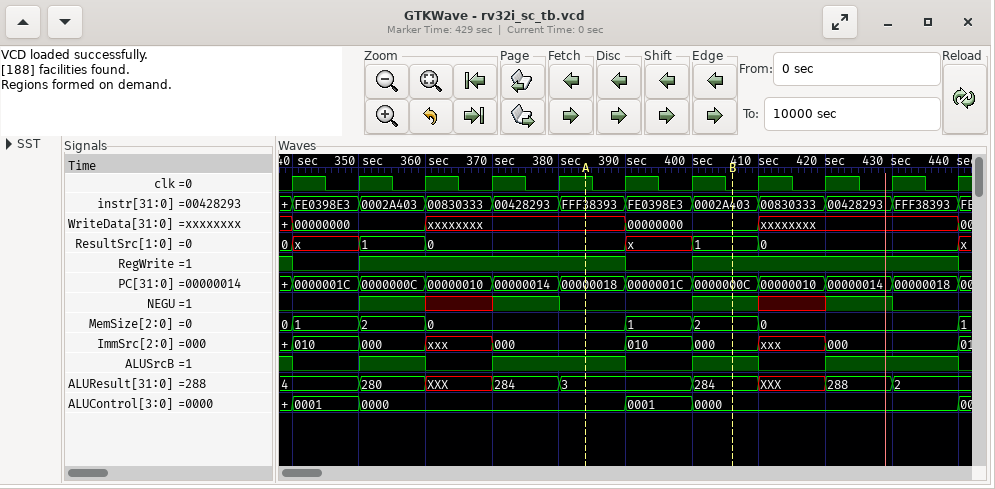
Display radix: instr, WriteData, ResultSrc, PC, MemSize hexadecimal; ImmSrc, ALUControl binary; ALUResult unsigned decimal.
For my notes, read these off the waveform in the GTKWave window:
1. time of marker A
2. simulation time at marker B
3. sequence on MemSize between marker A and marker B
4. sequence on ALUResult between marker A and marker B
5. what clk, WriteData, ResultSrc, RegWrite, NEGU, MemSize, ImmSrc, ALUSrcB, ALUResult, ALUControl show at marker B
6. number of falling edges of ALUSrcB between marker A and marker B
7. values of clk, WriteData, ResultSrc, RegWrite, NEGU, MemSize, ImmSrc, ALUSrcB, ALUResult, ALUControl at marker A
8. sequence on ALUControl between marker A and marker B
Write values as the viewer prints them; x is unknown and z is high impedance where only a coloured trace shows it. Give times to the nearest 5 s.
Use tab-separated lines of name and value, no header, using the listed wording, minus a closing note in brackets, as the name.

time of marker A	385 s
simulation time at marker B	405 s
sequence on MemSize between marker A and marker B	0, 1, 2
sequence on ALUResult between marker A and marker B	3, 284
what clk, WriteData, ResultSrc, RegWrite, NEGU, MemSize, ImmSrc, ALUSrcB, ALUResult, ALUControl show at marker B	clk=0, WriteData=00000000, ResultSrc=1, RegWrite=1, NEGU=1, MemSize=2, ImmSrc=000, ALUSrcB=1, ALUResult=284, ALUControl=0000
number of falling edges of ALUSrcB between marker A and marker B	1
values of clk, WriteData, ResultSrc, RegWrite, NEGU, MemSize, ImmSrc, ALUSrcB, ALUResult, ALUControl at marker A	clk=1, WriteData=xxxxxxxx, ResultSrc=0, RegWrite=1, NEGU=0, MemSize=0, ImmSrc=000, ALUSrcB=1, ALUResult=3, ALUControl=0000
sequence on ALUControl between marker A and marker B	0000, 0001, 0000
